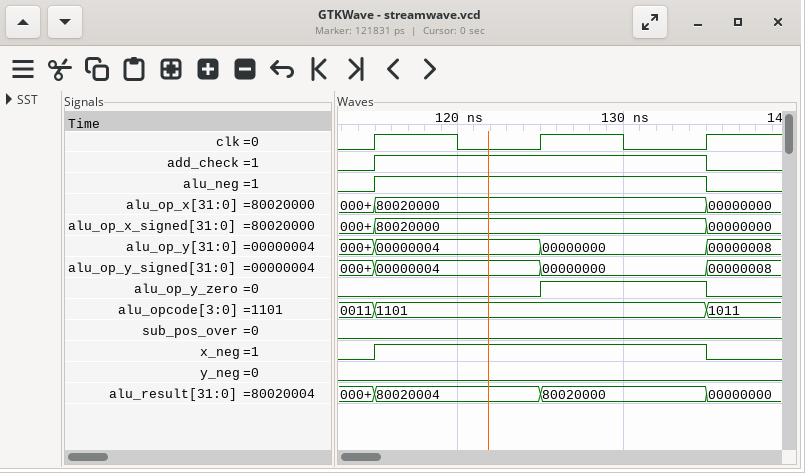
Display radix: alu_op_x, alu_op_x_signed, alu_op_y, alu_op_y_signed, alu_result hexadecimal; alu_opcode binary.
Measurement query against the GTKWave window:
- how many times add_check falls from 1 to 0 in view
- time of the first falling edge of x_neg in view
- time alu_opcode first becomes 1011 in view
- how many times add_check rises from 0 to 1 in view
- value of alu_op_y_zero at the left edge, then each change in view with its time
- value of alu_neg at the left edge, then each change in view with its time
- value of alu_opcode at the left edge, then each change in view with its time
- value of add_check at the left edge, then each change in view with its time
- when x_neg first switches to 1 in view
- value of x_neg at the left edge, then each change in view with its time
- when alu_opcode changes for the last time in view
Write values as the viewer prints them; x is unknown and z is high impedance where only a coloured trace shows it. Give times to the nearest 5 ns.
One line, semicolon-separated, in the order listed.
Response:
1; 135 ns; 135 ns; 1; 0, 1 at 125 ns, 0 at 135 ns; 0, 1 at 115 ns, 0 at 135 ns; 0011, 1101 at 115 ns, 1011 at 135 ns; 0, 1 at 115 ns, 0 at 135 ns; 115 ns; 0, 1 at 115 ns, 0 at 135 ns; 135 ns
